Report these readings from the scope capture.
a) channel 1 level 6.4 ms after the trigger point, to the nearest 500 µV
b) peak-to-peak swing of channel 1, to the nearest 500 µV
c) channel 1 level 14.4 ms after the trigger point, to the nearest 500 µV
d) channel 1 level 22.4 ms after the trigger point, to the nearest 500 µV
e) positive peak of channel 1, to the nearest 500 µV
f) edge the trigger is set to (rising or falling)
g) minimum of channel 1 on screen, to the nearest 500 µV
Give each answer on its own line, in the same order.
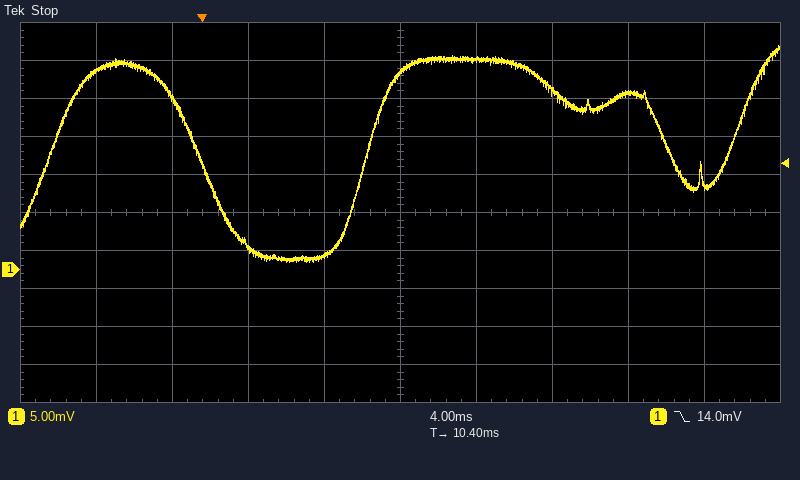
2.0 mV
28.5 mV
27.5 mV
23.0 mV
29.5 mV
falling
1.0 mV
